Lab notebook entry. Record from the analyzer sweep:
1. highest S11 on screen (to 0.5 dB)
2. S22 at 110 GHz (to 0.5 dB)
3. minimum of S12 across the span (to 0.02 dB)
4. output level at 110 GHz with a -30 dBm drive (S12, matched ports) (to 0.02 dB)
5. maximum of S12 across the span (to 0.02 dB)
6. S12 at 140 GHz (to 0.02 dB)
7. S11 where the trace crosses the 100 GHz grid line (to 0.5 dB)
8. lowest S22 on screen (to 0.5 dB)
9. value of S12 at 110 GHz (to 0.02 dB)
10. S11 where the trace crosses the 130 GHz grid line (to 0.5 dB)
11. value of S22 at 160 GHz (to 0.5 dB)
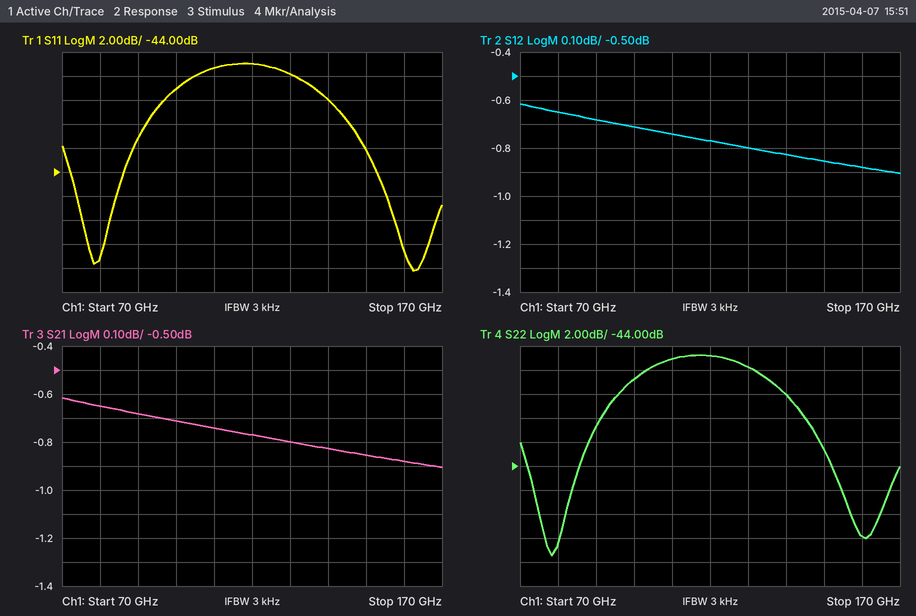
-35.0 dB
-35.0 dB
-0.90 dB
-30.74 dBm
-0.62 dB
-0.82 dB
-37.0 dB
-51.5 dB
-0.74 dB
-36.0 dB
-50.0 dB
